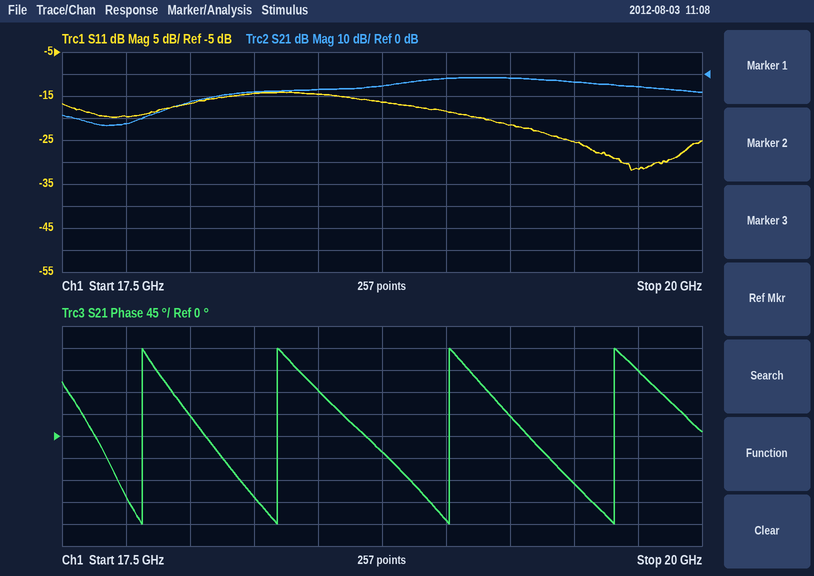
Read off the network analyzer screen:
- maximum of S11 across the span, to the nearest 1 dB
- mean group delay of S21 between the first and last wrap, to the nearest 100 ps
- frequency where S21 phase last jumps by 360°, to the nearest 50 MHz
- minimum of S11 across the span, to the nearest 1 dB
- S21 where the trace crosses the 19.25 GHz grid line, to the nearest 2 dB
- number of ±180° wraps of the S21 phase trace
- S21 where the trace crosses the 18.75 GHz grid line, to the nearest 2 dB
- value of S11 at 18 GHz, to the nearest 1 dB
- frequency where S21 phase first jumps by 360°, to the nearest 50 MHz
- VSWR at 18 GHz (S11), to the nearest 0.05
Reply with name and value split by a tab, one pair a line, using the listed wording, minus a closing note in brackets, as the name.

maximum of S11 across the span, to the nearest 1 dB	-14 dB
mean group delay of S21 between the first and last wrap, to the nearest 100 ps	1.6 ns
frequency where S21 phase last jumps by 360°, to the nearest 50 MHz	19.65 GHz
minimum of S11 across the span, to the nearest 1 dB	-32 dB
S21 where the trace crosses the 19.25 GHz grid line, to the nearest 2 dB	-2 dB
number of ±180° wraps of the S21 phase trace	4
S21 where the trace crosses the 18.75 GHz grid line, to the nearest 2 dB	-6 dB
value of S11 at 18 GHz, to the nearest 1 dB	-17 dB
frequency where S21 phase first jumps by 360°, to the nearest 50 MHz	17.80 GHz
VSWR at 18 GHz (S11), to the nearest 0.05	1.35
